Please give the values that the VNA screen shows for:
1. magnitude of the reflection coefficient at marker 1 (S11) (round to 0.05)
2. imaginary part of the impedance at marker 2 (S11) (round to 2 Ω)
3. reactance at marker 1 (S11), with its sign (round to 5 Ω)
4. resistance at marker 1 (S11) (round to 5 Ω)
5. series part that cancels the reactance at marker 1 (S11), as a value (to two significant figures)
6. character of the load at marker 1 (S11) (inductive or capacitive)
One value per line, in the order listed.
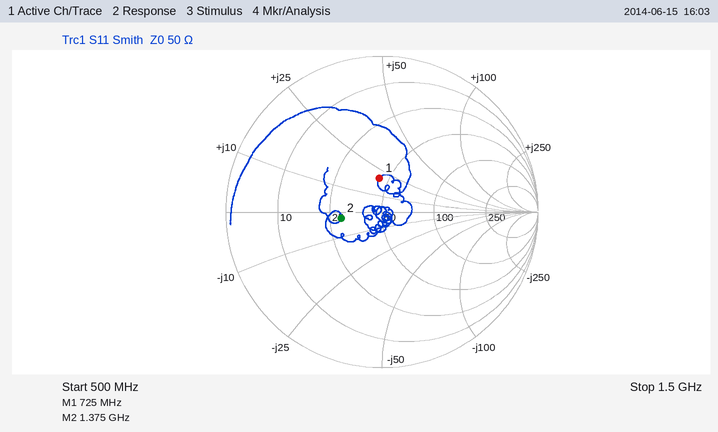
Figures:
0.20
-2 Ω
+20 Ω
45 Ω
11 pF
inductive
